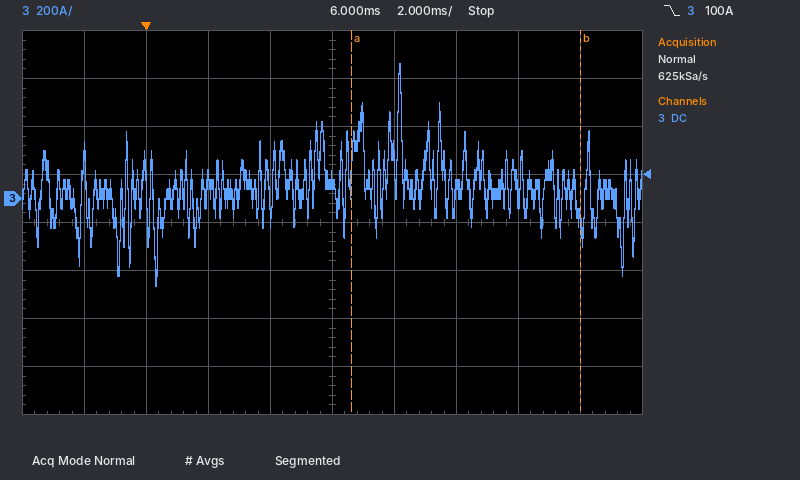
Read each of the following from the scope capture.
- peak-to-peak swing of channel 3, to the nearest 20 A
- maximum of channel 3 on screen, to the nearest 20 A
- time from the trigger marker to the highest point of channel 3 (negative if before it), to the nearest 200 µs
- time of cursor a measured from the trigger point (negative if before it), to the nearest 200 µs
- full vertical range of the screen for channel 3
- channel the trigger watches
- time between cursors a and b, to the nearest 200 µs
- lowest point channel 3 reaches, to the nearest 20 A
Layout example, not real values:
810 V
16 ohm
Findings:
920 A
560 A
+8.2 ms
+6.6 ms
1.6 kA
channel 3
7.4 ms
-360 A
